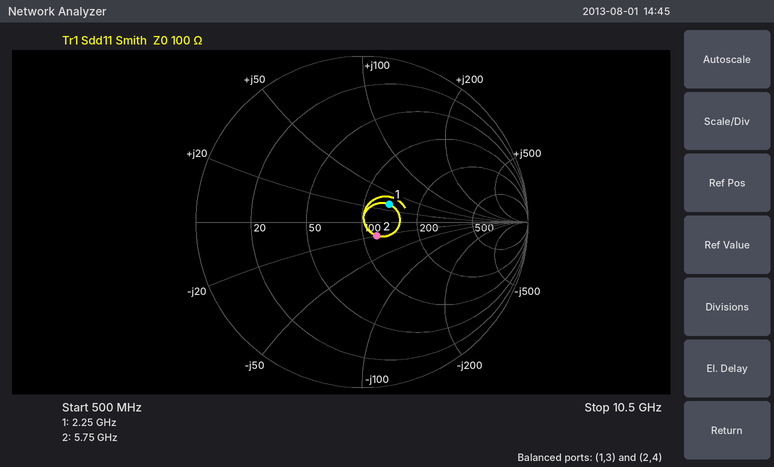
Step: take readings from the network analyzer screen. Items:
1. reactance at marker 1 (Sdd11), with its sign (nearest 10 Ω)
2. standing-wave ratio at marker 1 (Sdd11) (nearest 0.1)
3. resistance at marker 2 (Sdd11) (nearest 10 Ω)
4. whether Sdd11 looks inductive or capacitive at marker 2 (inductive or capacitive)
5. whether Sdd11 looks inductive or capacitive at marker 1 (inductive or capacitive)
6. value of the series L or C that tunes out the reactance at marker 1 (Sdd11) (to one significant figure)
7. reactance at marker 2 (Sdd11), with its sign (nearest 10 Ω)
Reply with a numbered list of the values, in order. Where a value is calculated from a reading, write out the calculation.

1. +30 Ω
2. 1.5
3. 120 Ω
4. capacitive
5. inductive
6. C = 1/(2π × 2.25 GHz × 30 Ω) ≈ 2 pF
7. -20 Ω
